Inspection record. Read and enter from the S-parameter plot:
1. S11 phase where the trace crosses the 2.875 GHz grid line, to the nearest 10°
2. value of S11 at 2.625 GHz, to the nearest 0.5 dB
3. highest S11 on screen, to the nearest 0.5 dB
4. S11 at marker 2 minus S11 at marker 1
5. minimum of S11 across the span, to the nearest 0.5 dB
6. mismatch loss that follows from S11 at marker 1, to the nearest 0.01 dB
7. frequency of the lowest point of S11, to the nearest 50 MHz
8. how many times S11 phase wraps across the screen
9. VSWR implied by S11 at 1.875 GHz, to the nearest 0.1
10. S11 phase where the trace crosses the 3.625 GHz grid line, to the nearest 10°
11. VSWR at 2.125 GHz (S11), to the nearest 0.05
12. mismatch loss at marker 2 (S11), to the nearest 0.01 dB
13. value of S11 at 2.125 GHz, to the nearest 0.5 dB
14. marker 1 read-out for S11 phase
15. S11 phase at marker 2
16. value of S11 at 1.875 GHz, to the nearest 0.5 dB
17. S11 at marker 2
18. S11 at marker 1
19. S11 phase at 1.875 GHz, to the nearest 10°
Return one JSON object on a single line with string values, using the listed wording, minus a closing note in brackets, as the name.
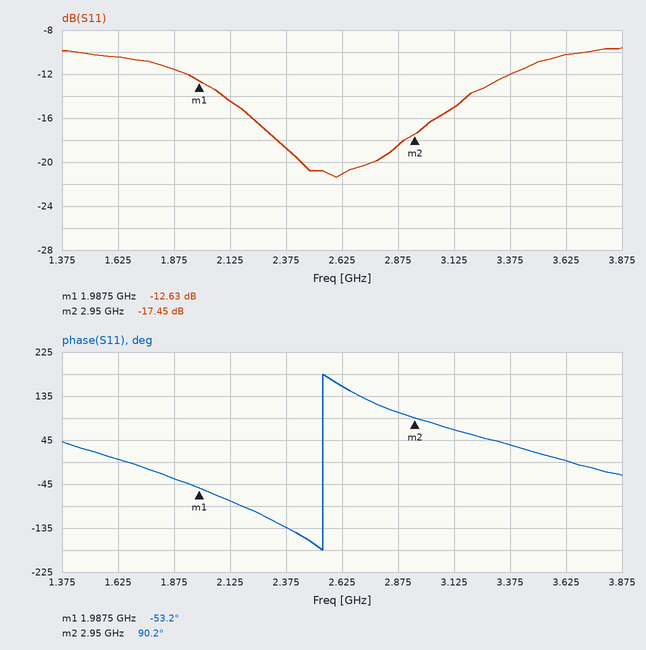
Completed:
{"S11 phase where the trace crosses the 2.875 GHz grid line, to the nearest 10°": "100°", "value of S11 at 2.625 GHz, to the nearest 0.5 dB": "-21.0 dB", "highest S11 on screen, to the nearest 0.5 dB": "-9.5 dB", "S11 at marker 2 minus S11 at marker 1": "-4.82 dB", "minimum of S11 across the span, to the nearest 0.5 dB": "-21.5 dB", "mismatch loss that follows from S11 at marker 1, to the nearest 0.01 dB": "0.24 dB", "frequency of the lowest point of S11, to the nearest 50 MHz": "2.60 GHz", "how many times S11 phase wraps across the screen": "1", "VSWR implied by S11 at 1.875 GHz, to the nearest 0.1": "1.7", "S11 phase where the trace crosses the 3.625 GHz grid line, to the nearest 10°": "0°", "VSWR at 2.125 GHz (S11), to the nearest 0.05": "1.45", "mismatch loss at marker 2 (S11), to the nearest 0.01 dB": "0.08 dB", "value of S11 at 2.125 GHz, to the nearest 0.5 dB": "-14.5 dB", "marker 1 read-out for S11 phase": "-53.2°", "S11 phase at marker 2": "90.2°", "value of S11 at 1.875 GHz, to the nearest 0.5 dB": "-11.5 dB", "S11 at marker 2": "-17.45 dB", "S11 at marker 1": "-12.63 dB", "S11 phase at 1.875 GHz, to the nearest 10°": "-30°"}
